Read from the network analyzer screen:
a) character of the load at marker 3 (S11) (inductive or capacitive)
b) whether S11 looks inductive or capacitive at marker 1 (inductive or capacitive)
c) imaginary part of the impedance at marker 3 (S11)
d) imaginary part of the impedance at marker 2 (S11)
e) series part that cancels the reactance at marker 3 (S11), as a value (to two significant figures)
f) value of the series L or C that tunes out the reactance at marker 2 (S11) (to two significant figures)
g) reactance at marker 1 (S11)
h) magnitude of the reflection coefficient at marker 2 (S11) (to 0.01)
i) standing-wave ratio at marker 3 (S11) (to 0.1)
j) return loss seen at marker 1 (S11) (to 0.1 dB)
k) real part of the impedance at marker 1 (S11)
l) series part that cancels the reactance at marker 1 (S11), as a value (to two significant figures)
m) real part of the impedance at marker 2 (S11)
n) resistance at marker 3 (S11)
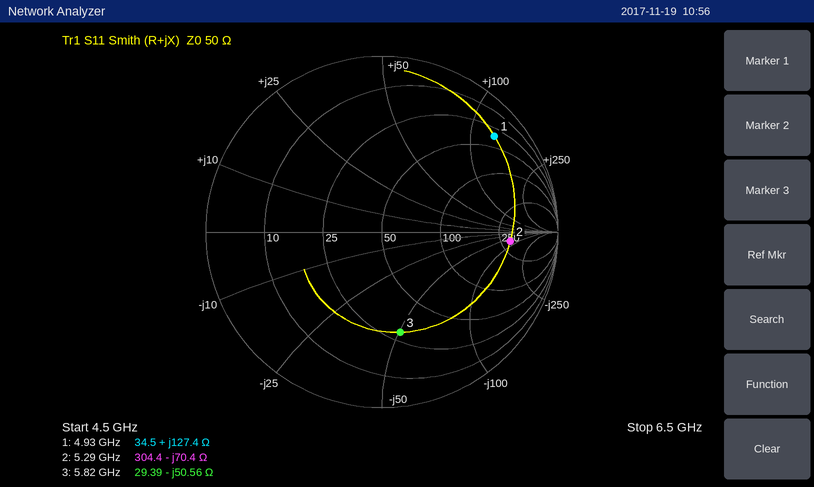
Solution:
capacitive
inductive
-50.56 Ω
-70.4 Ω
1.4 nH
2.1 nH
+127.4 Ω
0.73
3.8
1.5 dB
34.5 Ω
250 fF
304.4 Ω
29.39 Ω
